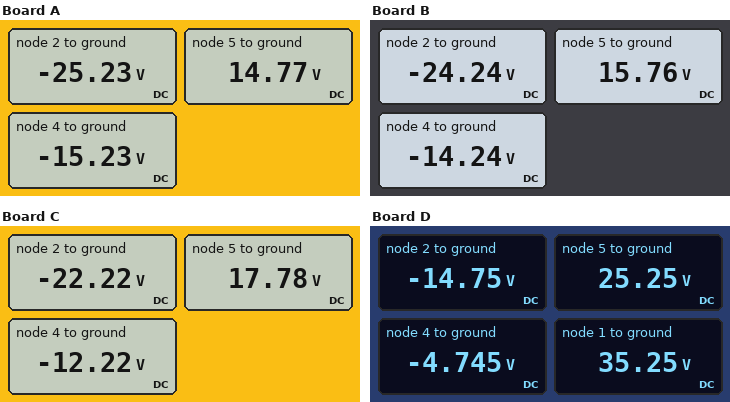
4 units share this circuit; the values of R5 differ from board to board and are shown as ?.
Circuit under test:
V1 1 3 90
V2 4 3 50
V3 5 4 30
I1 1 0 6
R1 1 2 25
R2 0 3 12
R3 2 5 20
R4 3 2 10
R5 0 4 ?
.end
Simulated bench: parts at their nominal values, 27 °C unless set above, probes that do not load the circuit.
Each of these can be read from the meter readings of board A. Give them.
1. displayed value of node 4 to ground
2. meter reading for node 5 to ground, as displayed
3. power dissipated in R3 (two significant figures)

-15.23 V
14.77 V
80 W
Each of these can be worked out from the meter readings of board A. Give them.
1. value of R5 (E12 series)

27 Ω
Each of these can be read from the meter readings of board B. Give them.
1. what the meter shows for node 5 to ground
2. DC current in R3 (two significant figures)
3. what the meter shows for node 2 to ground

15.76 V
2.0 A
-24.24 V
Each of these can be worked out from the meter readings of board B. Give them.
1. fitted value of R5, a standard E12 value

22 Ω
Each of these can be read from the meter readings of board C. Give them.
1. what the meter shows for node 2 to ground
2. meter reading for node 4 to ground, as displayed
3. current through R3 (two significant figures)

-22.22 V
-12.22 V
2.0 A
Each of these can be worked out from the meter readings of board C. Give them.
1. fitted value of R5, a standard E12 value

15 Ω
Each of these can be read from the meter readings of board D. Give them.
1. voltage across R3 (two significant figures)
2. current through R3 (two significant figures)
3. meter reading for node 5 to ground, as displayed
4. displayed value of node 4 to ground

40 V
2.0 A
25.25 V
-4.745 V
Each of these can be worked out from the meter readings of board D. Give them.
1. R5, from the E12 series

3.3 Ω
